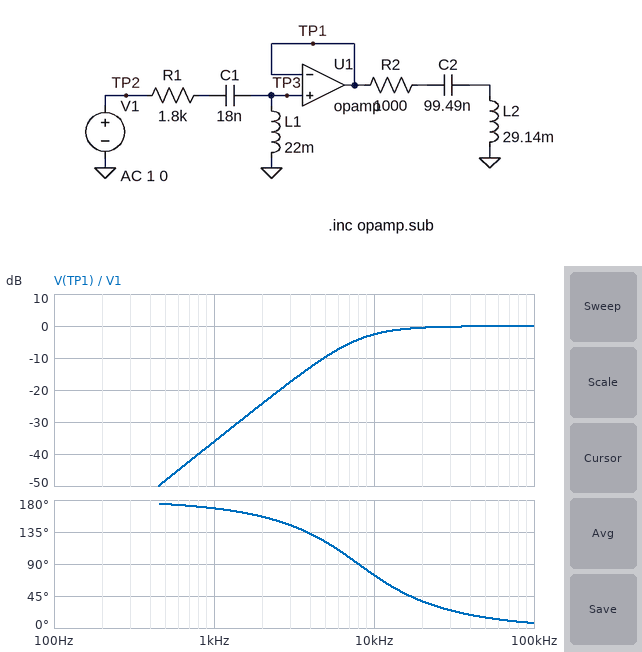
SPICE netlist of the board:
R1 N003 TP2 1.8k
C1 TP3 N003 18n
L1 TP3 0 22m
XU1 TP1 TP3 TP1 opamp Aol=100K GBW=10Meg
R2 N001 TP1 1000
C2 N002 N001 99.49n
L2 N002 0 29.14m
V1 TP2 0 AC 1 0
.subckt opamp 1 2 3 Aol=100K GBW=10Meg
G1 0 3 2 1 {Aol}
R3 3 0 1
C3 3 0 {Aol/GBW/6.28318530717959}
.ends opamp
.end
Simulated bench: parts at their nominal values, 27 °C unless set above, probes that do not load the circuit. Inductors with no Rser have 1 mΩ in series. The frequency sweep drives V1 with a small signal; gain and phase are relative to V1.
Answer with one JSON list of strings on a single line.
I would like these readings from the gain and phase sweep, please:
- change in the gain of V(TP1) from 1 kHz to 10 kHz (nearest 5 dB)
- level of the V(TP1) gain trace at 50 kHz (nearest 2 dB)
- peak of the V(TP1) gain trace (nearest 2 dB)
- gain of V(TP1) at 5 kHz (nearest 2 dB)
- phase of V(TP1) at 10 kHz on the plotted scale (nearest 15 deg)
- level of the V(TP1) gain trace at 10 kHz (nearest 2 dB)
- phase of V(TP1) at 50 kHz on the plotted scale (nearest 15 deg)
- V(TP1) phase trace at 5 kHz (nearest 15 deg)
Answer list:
["35 dB", "0 dB", "0 dB", "-10 dB", "75 deg", "-2 dB", "15 deg", "120 deg"]
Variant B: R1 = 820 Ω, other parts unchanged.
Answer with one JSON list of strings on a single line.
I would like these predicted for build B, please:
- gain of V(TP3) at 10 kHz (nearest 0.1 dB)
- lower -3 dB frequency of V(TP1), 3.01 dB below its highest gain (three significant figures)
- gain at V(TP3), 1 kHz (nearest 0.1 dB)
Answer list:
["3.2 dB", "6.73 kHz", "-36.0 dB"]
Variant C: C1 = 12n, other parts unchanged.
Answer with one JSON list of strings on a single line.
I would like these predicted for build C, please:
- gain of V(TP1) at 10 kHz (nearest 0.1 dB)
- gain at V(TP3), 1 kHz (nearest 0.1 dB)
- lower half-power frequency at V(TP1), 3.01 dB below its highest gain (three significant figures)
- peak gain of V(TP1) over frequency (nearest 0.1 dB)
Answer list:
["-2.3 dB", "-39.6 dB", "9.30 kHz", "0.1 dB"]
